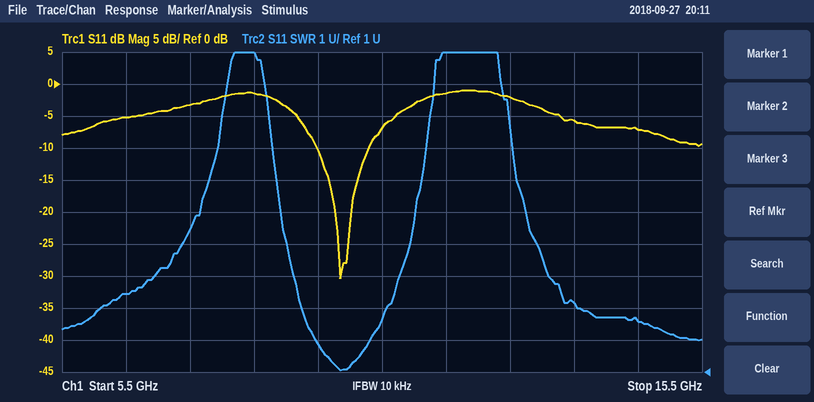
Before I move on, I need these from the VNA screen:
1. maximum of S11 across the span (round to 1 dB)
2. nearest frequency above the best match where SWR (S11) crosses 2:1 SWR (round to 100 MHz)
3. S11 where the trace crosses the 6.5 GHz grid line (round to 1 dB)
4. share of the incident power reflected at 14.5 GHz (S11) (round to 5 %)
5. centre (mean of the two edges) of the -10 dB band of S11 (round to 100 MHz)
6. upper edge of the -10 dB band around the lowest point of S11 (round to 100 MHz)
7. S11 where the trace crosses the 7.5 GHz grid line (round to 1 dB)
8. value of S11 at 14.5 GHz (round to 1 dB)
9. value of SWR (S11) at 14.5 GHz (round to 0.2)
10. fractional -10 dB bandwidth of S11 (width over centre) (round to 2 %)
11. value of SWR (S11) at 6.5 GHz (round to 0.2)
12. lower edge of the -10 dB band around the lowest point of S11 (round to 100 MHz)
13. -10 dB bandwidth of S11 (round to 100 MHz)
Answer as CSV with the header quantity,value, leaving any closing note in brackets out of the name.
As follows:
quantity,value
maximum of S11 across the span,-1 dB
nearest frequency above the best match where SWR (S11) crosses 2:1 SWR,10.3 GHz
S11 where the trace crosses the 6.5 GHz grid line,-5 dB
share of the incident power reflected at 14.5 GHz (S11),20 %
centre (mean of the two edges) of the -10 dB band of S11,9.9 GHz
upper edge of the -10 dB band around the lowest point of S11,10.3 GHz
S11 where the trace crosses the 7.5 GHz grid line,-3 dB
value of S11 at 14.5 GHz,-7 dB
value of SWR (S11) at 14.5 GHz,2.6
fractional -10 dB bandwidth of S11 (width over centre),8 %
value of SWR (S11) at 6.5 GHz,3.4
lower edge of the -10 dB band around the lowest point of S11,9.5 GHz
-10 dB bandwidth of S11,800 MHz
